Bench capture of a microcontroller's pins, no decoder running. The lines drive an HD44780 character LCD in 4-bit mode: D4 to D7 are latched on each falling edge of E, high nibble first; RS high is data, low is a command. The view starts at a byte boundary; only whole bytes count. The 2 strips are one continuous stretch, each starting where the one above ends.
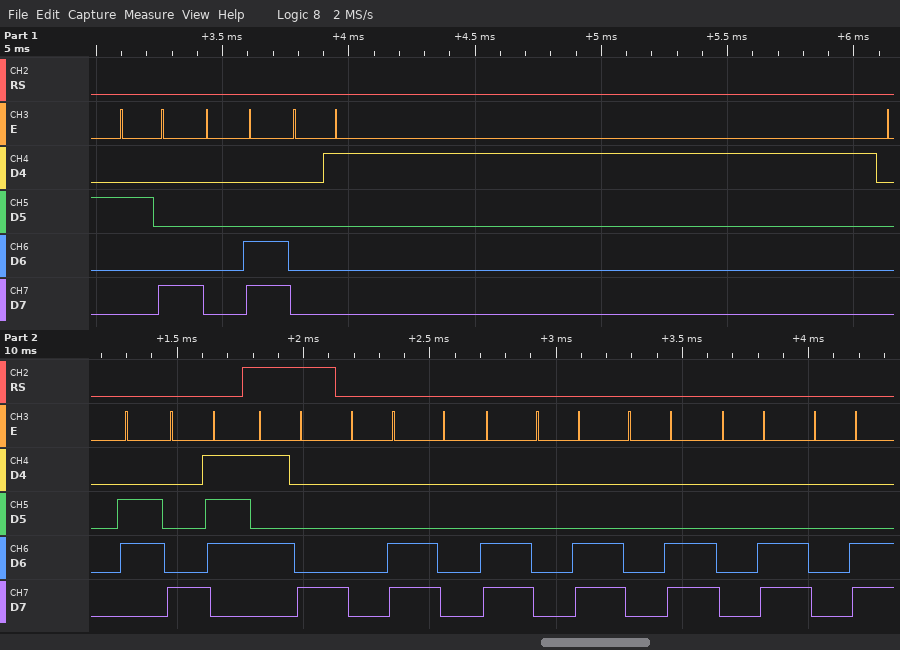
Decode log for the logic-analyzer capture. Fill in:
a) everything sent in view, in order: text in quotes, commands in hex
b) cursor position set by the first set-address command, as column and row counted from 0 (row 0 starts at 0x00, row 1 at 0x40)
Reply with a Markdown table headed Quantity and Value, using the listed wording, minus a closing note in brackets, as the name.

| Quantity | Value |
|---|---|
| everything sent in view, in order: text in quotes, commands in hex | 0x28 0x0C 0x01 0x06 0x87 "X" 0x0C 0x0C 0x0C 0x0C 0x0C 0x0C |
| cursor position set by the first set-address command, as column and row counted from 0 | column 7, row 0 |
